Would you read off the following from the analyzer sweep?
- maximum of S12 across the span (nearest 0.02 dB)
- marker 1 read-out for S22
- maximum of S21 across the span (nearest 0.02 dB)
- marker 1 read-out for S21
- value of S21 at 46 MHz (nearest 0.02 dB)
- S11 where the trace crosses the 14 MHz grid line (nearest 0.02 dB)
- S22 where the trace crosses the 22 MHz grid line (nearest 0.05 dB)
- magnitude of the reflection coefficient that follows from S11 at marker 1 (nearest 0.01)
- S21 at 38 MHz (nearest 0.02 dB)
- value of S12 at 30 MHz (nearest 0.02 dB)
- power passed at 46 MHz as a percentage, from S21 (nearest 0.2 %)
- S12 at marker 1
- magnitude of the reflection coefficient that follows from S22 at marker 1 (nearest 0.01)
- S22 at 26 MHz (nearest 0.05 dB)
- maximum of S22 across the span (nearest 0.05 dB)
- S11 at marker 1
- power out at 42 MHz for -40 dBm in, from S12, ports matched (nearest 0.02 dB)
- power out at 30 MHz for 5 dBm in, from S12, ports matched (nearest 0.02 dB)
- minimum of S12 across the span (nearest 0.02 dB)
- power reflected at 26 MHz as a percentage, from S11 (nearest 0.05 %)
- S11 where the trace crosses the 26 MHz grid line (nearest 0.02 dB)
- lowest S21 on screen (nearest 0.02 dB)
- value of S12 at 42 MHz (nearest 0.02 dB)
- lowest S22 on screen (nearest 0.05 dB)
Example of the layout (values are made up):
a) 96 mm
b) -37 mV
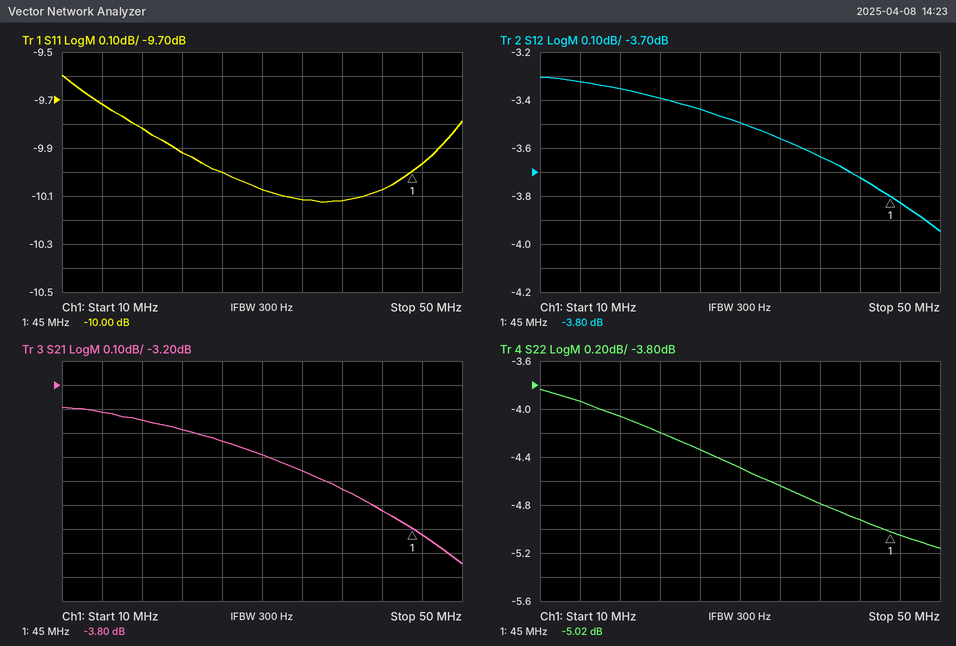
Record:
a) -3.30 dB
b) -5.02 dB
c) -3.30 dB
d) -3.80 dB
e) -3.82 dB
f) -9.72 dB
g) -4.20 dB
h) 0.32
i) -3.64 dB
j) -3.50 dB
k) 41.4 %
l) -3.80 dB
m) 0.56
n) -4.35 dB
o) -3.85 dB
p) -10.00 dB
q) -43.72 dBm
r) 1.50 dBm
s) -3.94 dB
t) 10.00 %
u) -10.00 dB
v) -3.94 dB
w) -3.72 dB
x) -5.15 dB
